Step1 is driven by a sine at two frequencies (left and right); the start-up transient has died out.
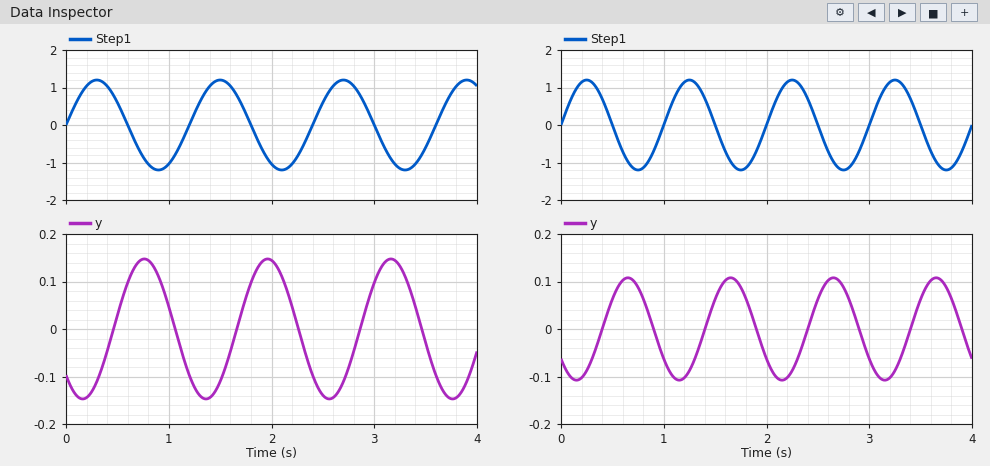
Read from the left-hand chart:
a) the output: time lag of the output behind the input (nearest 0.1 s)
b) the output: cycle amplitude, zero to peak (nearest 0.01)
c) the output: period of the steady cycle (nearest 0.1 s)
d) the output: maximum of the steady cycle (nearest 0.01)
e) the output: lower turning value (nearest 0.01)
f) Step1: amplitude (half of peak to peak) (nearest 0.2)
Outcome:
0.5 s
0.15
1.2 s
0.15
-0.15
1.2
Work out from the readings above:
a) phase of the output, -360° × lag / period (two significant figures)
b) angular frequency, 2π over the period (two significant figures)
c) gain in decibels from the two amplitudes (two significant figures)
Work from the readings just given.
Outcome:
-150°
5.2 rad/s
-18 dB
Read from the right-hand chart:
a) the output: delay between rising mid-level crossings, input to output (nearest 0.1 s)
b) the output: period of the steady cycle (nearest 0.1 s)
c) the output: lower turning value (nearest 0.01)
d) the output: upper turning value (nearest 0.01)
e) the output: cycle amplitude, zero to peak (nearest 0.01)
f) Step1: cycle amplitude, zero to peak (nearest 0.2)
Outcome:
0.4 s
1.0 s
-0.11
0.11
0.11
1.2
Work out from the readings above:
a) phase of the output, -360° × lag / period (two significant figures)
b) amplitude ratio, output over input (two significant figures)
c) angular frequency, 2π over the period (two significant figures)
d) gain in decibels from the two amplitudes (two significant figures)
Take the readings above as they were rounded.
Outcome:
-140°
0.092
6.3 rad/s
-21 dB
